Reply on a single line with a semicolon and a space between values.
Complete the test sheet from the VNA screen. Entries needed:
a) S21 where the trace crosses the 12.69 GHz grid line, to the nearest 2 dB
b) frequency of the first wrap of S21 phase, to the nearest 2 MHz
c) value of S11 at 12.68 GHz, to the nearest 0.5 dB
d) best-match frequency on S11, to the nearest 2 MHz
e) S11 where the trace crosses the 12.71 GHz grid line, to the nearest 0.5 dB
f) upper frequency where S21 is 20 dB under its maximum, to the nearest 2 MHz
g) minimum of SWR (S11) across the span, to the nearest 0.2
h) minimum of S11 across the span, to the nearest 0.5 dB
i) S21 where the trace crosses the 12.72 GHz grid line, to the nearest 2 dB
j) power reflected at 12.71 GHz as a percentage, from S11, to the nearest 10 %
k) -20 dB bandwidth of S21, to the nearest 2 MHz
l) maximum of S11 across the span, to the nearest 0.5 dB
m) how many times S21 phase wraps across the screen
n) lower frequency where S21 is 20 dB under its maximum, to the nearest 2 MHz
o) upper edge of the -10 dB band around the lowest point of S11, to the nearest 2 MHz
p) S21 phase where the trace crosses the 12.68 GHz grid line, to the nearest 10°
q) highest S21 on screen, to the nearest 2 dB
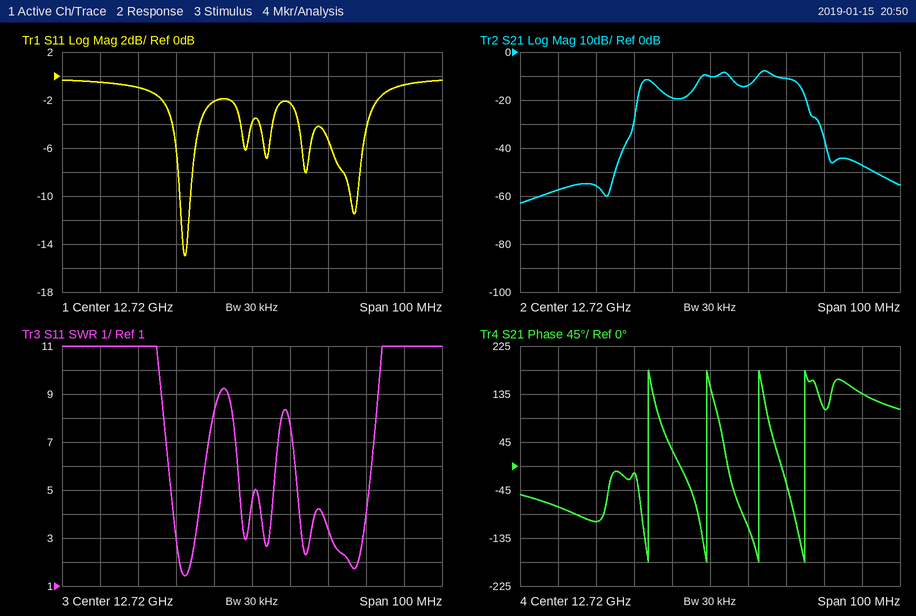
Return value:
-56 dB; 12.704 GHz; -0.5 dB; 12.702 GHz; -2.0 dB; 12.748 GHz; 1.4; -15.0 dB; -10 dB; 60 %; 48 MHz; -0.5 dB; 4; 12.700 GHz; 12.704 GHz; -80°; -8 dB
